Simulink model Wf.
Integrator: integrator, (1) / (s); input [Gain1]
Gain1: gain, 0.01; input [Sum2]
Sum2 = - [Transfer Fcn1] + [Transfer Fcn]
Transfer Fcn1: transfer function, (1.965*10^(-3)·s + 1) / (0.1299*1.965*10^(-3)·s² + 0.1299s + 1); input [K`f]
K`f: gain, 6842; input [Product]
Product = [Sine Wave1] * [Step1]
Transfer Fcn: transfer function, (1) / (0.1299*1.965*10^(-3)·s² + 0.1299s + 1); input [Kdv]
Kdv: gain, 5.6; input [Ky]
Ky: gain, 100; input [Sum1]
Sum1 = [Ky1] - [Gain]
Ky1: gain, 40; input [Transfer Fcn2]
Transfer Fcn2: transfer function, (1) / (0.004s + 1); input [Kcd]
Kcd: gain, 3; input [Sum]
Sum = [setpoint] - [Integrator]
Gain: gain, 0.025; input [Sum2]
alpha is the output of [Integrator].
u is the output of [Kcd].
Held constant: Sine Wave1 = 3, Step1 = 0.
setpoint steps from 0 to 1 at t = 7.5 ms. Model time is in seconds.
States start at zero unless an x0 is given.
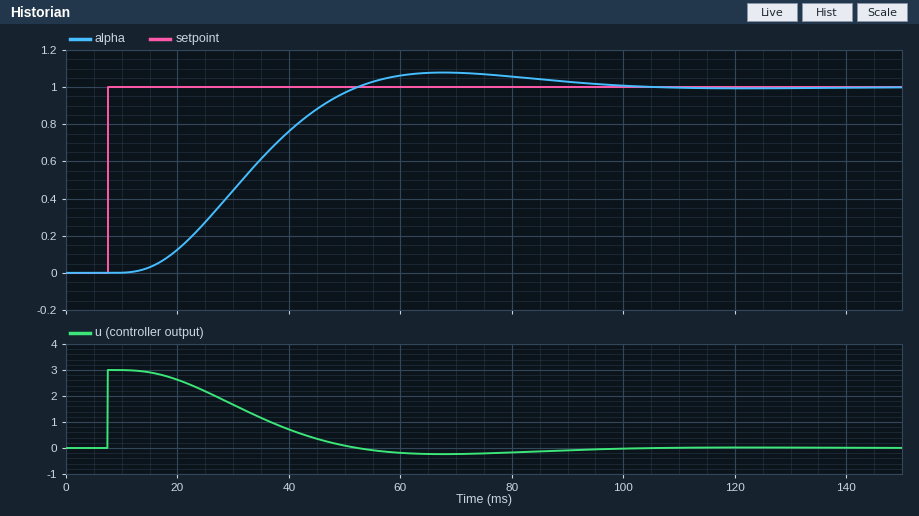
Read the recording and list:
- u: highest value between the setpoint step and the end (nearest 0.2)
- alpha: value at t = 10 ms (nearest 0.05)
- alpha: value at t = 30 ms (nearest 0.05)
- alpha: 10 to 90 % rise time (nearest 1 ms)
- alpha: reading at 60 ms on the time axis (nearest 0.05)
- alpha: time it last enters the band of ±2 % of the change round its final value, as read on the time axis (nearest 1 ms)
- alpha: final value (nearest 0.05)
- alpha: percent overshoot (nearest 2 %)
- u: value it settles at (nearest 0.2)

3.0
0.00
0.45
27 ms
1.05
94 ms
1.00
8 %
0.0
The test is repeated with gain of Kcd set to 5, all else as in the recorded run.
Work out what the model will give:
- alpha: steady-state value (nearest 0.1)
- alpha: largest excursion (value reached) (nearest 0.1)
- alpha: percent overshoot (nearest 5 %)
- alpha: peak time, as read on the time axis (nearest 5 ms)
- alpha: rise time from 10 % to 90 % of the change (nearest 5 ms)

1.0
1.3
25 %
50 ms
15 ms
